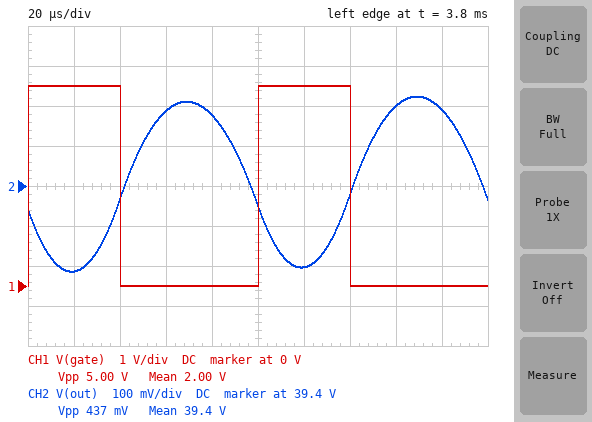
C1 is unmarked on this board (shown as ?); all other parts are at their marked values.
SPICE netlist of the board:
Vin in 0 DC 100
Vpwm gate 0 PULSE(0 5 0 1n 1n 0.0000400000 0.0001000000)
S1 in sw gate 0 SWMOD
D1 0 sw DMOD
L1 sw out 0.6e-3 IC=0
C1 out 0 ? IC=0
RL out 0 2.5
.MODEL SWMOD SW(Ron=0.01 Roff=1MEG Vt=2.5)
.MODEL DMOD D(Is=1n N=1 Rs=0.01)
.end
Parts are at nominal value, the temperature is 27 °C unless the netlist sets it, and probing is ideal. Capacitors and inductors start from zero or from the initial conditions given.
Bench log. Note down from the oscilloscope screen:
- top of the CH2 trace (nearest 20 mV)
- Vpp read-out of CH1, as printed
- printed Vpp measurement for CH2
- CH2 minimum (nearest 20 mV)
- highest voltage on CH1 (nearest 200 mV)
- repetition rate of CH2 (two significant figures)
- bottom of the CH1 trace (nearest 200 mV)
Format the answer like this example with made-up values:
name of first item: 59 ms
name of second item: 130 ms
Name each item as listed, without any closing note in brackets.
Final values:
top of the CH2 trace: 39.62 V
Vpp read-out of CH1, as printed: 5.00 V
printed Vpp measurement for CH2: 437 mV
CH2 minimum: 39.18 V
highest voltage on CH1: 5.0 V
repetition rate of CH2: 10 kHz
bottom of the CH1 trace: 0 V
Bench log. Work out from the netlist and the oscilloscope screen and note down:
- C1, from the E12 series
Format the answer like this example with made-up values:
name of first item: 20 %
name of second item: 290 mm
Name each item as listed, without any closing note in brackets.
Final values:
C1, from the E12 series: 120 µF
